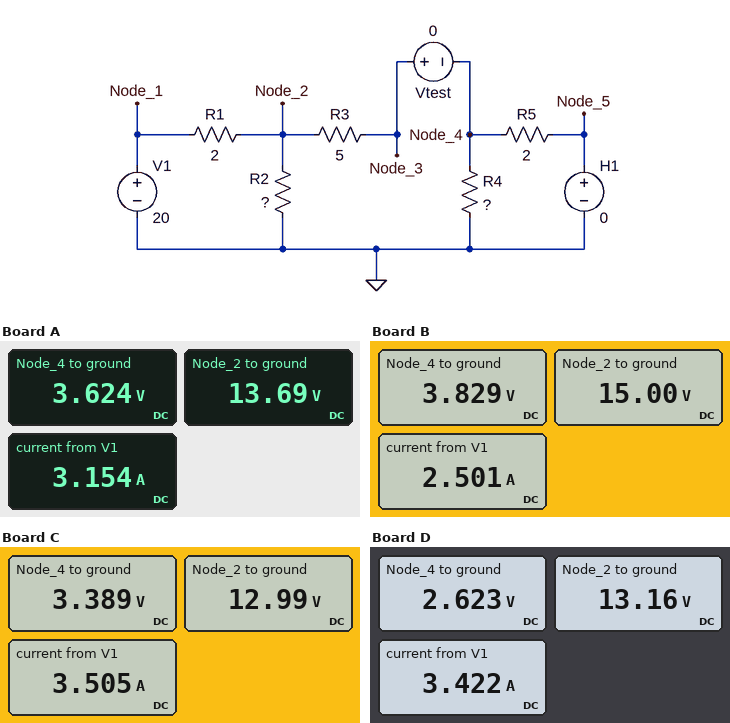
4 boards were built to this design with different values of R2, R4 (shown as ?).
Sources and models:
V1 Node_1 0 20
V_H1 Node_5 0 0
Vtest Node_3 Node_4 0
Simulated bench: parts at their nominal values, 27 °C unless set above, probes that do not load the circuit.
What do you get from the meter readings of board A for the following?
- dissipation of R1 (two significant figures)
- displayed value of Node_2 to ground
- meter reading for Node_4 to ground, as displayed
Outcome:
20 W
13.69 V
3.624 V
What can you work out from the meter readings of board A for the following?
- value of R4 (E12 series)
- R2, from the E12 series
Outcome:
18 Ω
12 Ω
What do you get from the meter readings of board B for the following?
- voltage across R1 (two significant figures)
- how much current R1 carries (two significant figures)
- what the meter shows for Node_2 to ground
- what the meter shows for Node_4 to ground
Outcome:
5.0 V
2.5 A
15.00 V
3.829 V
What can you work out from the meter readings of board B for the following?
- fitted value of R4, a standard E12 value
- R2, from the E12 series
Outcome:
12 Ω
56 Ω
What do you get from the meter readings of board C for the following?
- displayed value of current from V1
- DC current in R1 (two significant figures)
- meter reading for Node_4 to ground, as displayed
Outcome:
3.505 A
3.5 A
3.389 V
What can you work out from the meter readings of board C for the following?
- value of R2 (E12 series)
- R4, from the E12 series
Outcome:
8.2 Ω
15 Ω
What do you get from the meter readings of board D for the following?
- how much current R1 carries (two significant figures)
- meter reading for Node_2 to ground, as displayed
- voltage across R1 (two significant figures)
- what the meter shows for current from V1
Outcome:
3.4 A
13.16 V
6.8 V
3.422 A
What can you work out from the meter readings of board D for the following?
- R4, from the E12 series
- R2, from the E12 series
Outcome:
3.3 Ω
10 Ω
